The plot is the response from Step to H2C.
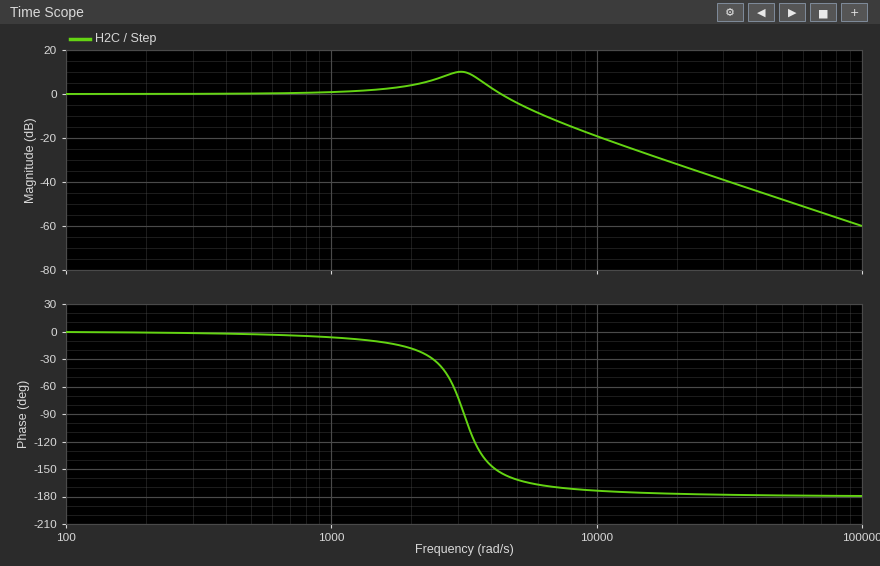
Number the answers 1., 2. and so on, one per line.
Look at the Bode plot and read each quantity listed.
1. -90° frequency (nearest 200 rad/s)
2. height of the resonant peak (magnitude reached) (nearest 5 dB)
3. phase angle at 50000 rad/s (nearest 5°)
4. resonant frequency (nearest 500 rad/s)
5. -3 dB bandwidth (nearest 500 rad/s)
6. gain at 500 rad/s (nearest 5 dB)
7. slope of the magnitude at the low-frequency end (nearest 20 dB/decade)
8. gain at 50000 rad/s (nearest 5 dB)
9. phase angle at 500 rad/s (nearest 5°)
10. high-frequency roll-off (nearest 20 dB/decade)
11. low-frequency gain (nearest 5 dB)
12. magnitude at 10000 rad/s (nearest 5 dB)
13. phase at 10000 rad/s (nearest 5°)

1. 3200 rad/s
2. 10 dB
3. -180°
4. 3000 rad/s
5. 5000 rad/s
6. 0 dB
7. 0 dB/decade
8. -50 dB
9. -5°
10. -40 dB/decade
11. 0 dB
12. -20 dB
13. -175°
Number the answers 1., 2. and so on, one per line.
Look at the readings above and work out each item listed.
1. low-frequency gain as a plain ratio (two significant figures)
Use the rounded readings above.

1. 1.0
